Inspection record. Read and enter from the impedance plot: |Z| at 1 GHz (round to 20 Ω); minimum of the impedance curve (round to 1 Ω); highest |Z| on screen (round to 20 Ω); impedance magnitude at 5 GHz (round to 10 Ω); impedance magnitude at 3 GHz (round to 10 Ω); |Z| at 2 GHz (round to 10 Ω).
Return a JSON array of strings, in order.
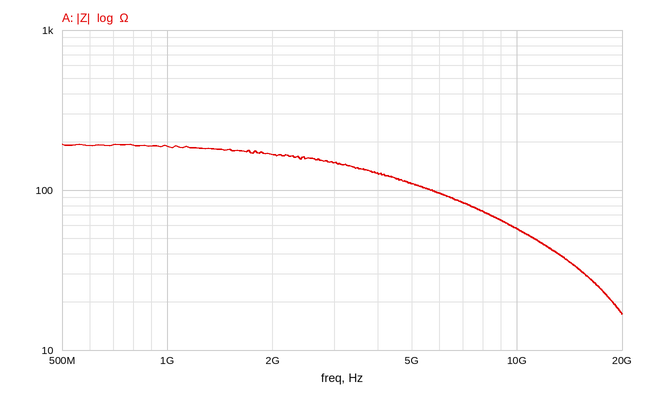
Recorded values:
["180 Ω", "17 Ω", "200 Ω", "110 Ω", "150 Ω", "170 Ω"]
